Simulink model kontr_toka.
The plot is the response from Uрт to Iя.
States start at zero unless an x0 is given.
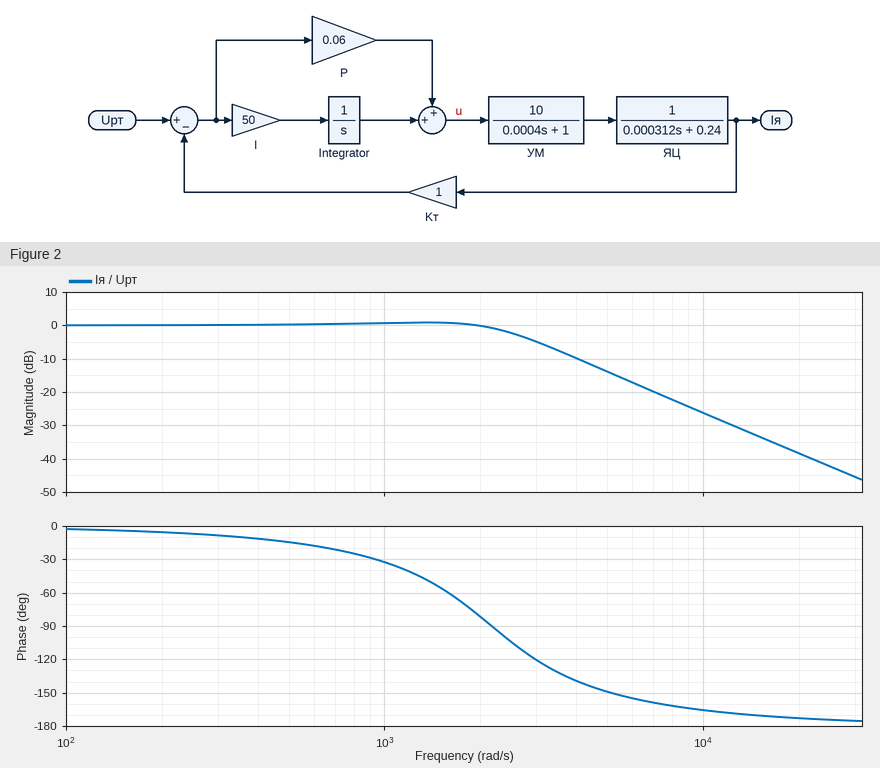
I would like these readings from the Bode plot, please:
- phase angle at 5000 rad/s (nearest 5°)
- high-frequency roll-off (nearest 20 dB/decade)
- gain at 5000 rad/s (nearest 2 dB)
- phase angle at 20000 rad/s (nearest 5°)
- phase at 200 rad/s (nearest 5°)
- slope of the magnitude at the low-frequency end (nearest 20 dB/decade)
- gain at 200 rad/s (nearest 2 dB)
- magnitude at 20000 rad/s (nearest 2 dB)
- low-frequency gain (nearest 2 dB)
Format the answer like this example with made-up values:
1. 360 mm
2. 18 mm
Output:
1. -150°
2. -40 dB/decade
3. -14 dB
4. -175°
5. -5°
6. 0 dB/decade
7. 0 dB
8. -38 dB
9. 0 dB
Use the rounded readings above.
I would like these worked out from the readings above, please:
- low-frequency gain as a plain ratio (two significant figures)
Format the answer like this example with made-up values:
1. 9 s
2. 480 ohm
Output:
1. 1.0
